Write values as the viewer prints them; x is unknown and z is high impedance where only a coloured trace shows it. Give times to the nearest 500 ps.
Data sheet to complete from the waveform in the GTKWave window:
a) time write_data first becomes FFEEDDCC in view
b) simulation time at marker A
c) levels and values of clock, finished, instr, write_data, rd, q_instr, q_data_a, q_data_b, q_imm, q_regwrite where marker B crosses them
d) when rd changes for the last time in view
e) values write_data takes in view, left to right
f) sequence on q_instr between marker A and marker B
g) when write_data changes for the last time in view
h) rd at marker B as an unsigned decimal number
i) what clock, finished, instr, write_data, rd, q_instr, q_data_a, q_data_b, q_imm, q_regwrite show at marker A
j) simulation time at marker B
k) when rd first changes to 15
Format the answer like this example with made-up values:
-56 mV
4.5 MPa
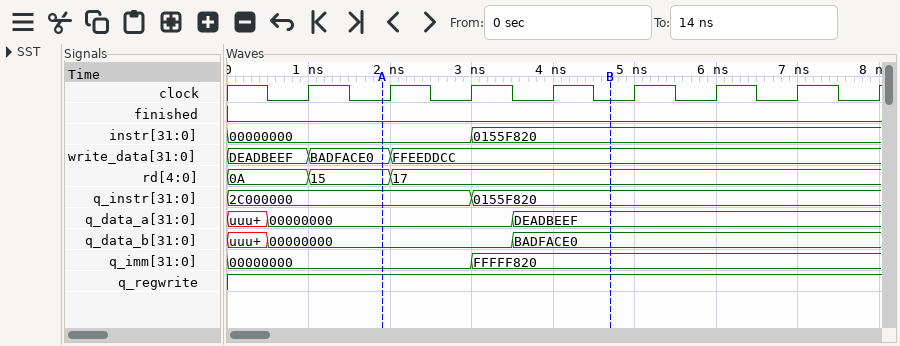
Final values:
2000 ps
2000 ps
clock=0, finished=0, instr=0155F820, write_data=FFEEDDCC, rd=17, q_instr=0155F820, q_data_a=DEADBEEF, q_data_b=BADFACE0, q_imm=FFFFF820, q_regwrite=1
2000 ps
DEADBEEF, BADFACE0, FFEEDDCC
2C000000, 0155F820
2000 ps
23
clock=0, finished=0, instr=00000000, write_data=BADFACE0, rd=15, q_instr=2C000000, q_data_a=00000000, q_data_b=00000000, q_imm=00000000, q_regwrite=1
4500 ps
1000 ps
